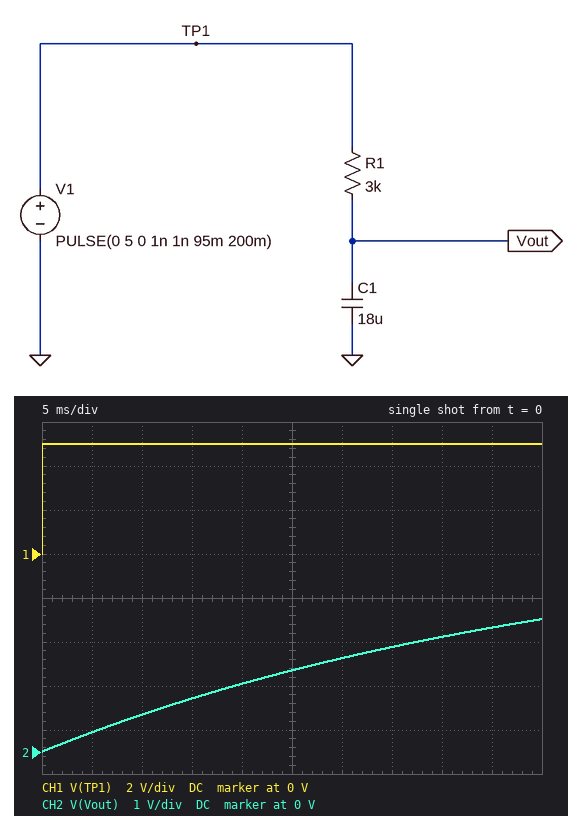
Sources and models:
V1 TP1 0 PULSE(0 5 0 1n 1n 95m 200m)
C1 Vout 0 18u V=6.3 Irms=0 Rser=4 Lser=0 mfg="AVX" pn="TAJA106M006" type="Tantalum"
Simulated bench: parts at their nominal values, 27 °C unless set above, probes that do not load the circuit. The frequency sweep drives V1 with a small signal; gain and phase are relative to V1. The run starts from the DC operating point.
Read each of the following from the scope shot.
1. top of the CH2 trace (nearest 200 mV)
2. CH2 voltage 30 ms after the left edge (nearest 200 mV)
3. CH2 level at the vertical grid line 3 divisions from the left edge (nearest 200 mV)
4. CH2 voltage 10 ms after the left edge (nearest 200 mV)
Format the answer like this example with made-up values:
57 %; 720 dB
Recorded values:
3.0 V; 2.2 V; 1.2 V; 800 mV
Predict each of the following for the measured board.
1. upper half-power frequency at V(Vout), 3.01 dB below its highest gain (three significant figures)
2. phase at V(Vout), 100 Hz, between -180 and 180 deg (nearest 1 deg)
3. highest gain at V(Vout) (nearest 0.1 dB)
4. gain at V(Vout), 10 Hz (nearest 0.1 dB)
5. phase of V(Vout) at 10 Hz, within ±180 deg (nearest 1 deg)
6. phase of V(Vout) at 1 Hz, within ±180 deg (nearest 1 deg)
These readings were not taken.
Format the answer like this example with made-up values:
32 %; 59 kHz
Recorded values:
2.94 Hz; -86 deg; 0 dB; -11.0 dB; -73 deg; -19 deg
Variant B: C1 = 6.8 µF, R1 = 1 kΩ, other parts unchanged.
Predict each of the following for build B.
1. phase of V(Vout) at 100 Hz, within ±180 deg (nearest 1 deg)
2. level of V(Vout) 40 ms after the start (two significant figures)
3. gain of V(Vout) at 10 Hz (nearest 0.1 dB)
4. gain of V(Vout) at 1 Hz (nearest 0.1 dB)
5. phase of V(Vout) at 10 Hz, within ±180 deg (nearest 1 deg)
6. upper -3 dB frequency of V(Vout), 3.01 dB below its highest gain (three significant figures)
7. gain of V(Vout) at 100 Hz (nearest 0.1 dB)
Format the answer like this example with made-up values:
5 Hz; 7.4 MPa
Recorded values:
-76 deg; 5.0 V; -0.7 dB; 0 dB; -23 deg; 23.3 Hz; -12.9 dB
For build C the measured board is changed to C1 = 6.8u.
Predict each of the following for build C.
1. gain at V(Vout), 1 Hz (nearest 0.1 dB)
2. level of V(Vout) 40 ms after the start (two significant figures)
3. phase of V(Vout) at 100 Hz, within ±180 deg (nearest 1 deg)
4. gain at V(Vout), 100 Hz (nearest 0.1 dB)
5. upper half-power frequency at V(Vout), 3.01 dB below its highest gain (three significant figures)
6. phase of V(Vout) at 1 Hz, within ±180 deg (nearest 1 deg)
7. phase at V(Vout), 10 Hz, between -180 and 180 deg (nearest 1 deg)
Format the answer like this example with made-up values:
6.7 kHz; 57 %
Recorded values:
-0.1 dB; 4.3 V; -85 deg; -22.2 dB; 7.79 Hz; -7 deg; -52 deg
